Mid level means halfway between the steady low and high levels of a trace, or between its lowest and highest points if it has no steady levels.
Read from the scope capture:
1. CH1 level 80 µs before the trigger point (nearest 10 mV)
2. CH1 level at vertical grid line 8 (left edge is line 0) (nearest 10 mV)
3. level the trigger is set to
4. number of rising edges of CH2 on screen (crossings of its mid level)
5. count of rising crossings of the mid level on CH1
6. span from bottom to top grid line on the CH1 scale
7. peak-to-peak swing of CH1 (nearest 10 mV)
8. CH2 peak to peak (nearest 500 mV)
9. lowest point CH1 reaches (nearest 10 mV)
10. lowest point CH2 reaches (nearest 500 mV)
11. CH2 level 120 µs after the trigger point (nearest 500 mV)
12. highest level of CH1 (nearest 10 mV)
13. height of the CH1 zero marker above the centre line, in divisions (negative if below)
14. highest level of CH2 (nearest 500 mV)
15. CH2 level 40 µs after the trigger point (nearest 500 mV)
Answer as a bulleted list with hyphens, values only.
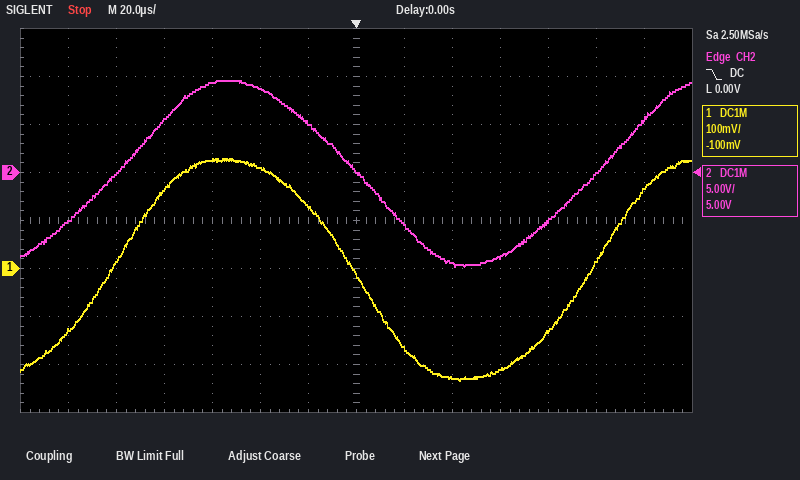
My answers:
- 160 mV
- -170 mV
- 0.00 V
- 2
- 2
- 800 mV
- 460 mV
- 19.5 V
- -230 mV
- -10.0 V
- 5.5 V
- 230 mV
- -1.0 div
- 9.5 V
- -9.5 V
